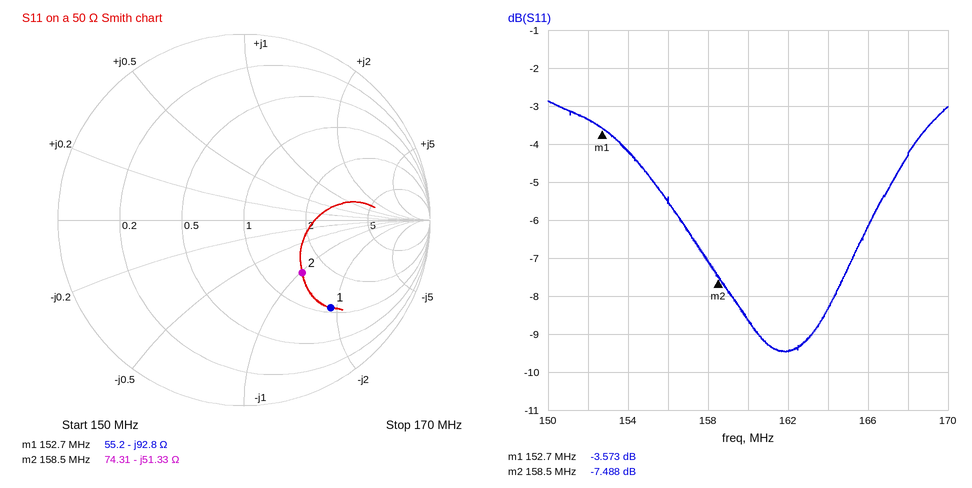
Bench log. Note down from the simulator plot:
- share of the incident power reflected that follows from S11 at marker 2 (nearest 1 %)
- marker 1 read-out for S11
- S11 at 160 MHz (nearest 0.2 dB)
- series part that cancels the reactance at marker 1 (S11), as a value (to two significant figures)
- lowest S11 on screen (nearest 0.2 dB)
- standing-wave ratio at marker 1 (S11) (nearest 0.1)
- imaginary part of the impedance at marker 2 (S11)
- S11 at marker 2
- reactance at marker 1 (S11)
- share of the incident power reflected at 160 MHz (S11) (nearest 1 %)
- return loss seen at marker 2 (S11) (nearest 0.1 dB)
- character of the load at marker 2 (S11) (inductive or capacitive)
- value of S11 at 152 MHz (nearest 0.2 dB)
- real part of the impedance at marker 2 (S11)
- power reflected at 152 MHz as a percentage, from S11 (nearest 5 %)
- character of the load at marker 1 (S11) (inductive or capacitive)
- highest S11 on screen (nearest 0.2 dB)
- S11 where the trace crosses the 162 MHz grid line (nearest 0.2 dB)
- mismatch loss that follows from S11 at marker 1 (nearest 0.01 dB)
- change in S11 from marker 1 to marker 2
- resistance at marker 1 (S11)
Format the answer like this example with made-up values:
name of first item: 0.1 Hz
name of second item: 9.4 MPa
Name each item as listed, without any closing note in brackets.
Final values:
share of the incident power reflected that follows from S11 at marker 2: 18 %
marker 1 read-out for S11: -3.573 dB
S11 at 160 MHz: -8.6 dB
series part that cancels the reactance at marker 1 (S11), as a value: 97 nH
lowest S11 on screen: -9.4 dB
standing-wave ratio at marker 1 (S11): 4.9
imaginary part of the impedance at marker 2: -51.33 Ω
S11 at marker 2: -7.488 dB
reactance at marker 1: -92.8 Ω
share of the incident power reflected at 160 MHz (S11): 14 %
return loss seen at marker 2 (S11): 7.5 dB
character of the load at marker 2 (S11): capacitive
value of S11 at 152 MHz: -3.4 dB
real part of the impedance at marker 2: 74.31 Ω
power reflected at 152 MHz as a percentage, from S11: 45 %
character of the load at marker 1 (S11): capacitive
highest S11 on screen: -2.8 dB
S11 where the trace crosses the 162 MHz grid line: -9.4 dB
mismatch loss that follows from S11 at marker 1: 2.51 dB
change in S11 from marker 1 to marker 2: -3.915 dB
resistance at marker 1: 55.2 Ω
